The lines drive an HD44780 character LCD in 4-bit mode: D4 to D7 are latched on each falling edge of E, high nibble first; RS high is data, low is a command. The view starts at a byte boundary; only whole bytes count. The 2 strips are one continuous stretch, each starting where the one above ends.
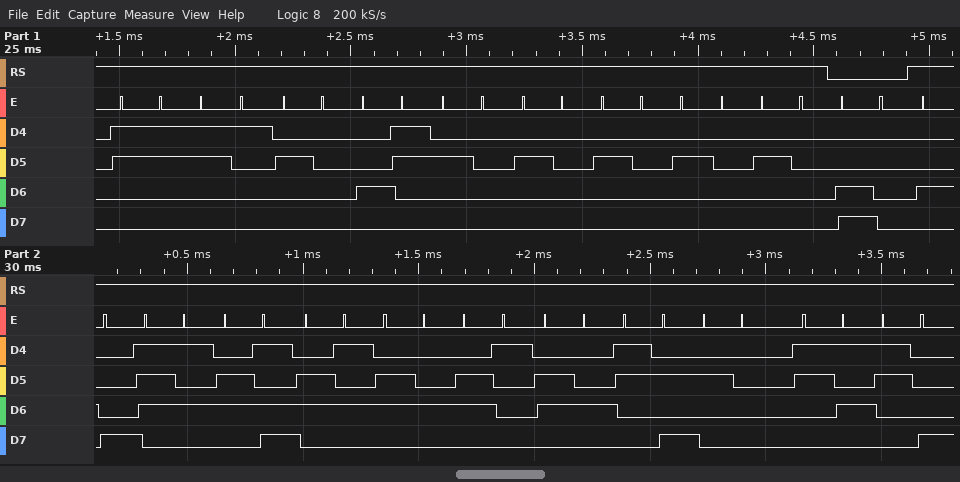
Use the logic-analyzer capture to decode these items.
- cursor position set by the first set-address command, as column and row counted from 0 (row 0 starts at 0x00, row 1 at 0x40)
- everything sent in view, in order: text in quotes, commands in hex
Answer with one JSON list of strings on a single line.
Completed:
["column 0, row 1", "\"31 C     \" 0xC0 \"Humedad: 58\""]
